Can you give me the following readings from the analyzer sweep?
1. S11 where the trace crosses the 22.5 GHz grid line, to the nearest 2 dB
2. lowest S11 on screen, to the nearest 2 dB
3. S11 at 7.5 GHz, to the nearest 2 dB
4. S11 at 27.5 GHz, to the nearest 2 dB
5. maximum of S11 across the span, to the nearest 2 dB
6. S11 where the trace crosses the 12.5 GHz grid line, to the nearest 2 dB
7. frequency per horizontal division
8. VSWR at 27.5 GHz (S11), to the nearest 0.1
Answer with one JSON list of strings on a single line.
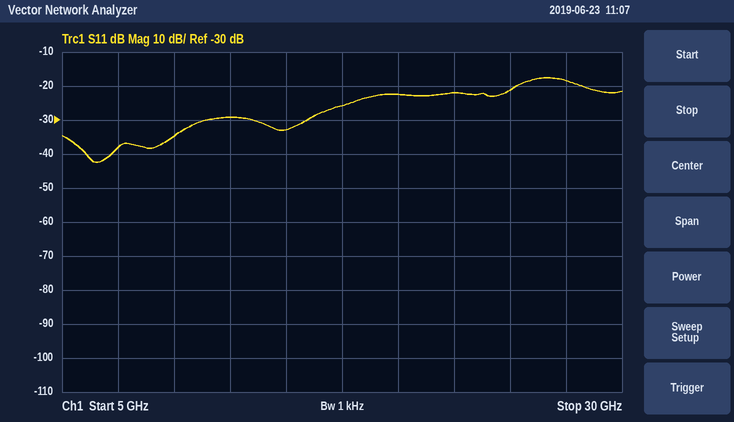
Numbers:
["-22 dB", "-42 dB", "-38 dB", "-18 dB", "-18 dB", "-30 dB", "2.5 GHz", "1.3"]
